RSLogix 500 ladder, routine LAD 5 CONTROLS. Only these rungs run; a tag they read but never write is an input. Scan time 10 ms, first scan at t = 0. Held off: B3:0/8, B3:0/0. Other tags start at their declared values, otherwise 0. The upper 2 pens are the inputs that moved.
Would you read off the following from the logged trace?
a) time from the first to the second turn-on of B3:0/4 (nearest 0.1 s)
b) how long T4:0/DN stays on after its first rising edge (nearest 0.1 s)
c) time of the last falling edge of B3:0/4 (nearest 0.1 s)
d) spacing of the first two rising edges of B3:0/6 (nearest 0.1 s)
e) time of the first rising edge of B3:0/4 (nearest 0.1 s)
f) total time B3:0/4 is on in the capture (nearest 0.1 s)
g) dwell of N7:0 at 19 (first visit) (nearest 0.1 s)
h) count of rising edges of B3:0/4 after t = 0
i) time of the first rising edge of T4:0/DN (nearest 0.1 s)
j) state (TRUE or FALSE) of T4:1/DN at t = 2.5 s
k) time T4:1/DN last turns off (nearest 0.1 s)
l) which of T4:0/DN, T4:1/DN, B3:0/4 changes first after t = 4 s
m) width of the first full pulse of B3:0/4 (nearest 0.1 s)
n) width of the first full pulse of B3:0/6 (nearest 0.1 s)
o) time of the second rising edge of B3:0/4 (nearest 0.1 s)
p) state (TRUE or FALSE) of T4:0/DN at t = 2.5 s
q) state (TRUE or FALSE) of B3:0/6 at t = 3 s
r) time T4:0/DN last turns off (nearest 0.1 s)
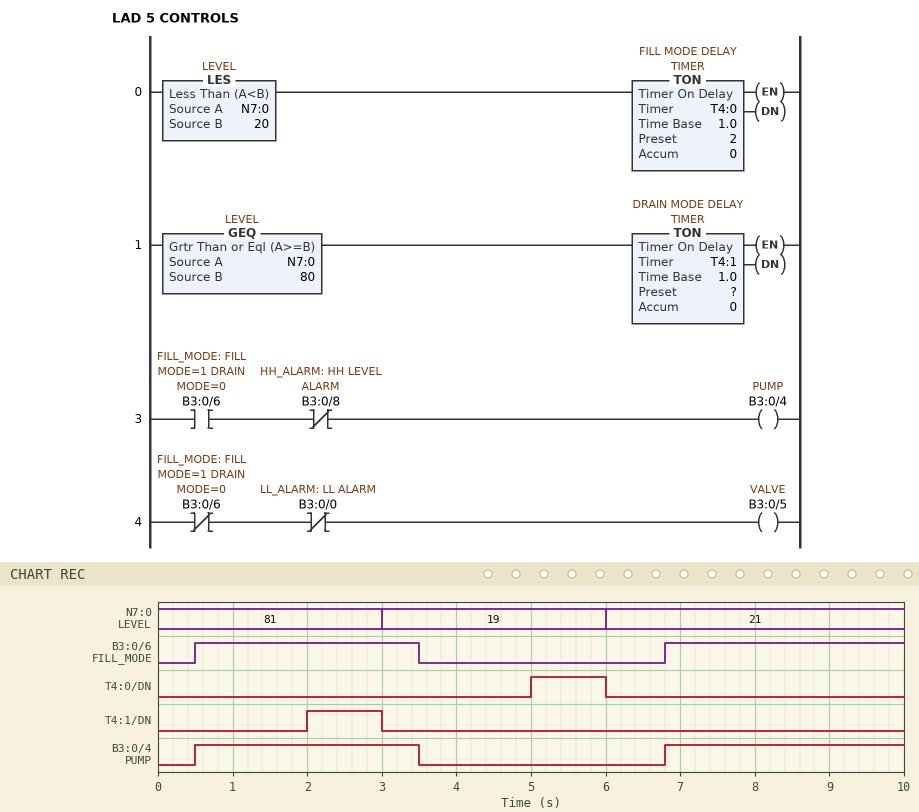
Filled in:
6.3 s
1.0 s
3.5 s
6.3 s
0.5 s
6.2 s
3.0 s
2
5.0 s
TRUE
3.0 s
T4:0/DN
3.0 s
3.0 s
6.8 s
FALSE
TRUE
6.0 s
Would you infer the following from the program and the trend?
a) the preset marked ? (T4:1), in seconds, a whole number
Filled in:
2 s
